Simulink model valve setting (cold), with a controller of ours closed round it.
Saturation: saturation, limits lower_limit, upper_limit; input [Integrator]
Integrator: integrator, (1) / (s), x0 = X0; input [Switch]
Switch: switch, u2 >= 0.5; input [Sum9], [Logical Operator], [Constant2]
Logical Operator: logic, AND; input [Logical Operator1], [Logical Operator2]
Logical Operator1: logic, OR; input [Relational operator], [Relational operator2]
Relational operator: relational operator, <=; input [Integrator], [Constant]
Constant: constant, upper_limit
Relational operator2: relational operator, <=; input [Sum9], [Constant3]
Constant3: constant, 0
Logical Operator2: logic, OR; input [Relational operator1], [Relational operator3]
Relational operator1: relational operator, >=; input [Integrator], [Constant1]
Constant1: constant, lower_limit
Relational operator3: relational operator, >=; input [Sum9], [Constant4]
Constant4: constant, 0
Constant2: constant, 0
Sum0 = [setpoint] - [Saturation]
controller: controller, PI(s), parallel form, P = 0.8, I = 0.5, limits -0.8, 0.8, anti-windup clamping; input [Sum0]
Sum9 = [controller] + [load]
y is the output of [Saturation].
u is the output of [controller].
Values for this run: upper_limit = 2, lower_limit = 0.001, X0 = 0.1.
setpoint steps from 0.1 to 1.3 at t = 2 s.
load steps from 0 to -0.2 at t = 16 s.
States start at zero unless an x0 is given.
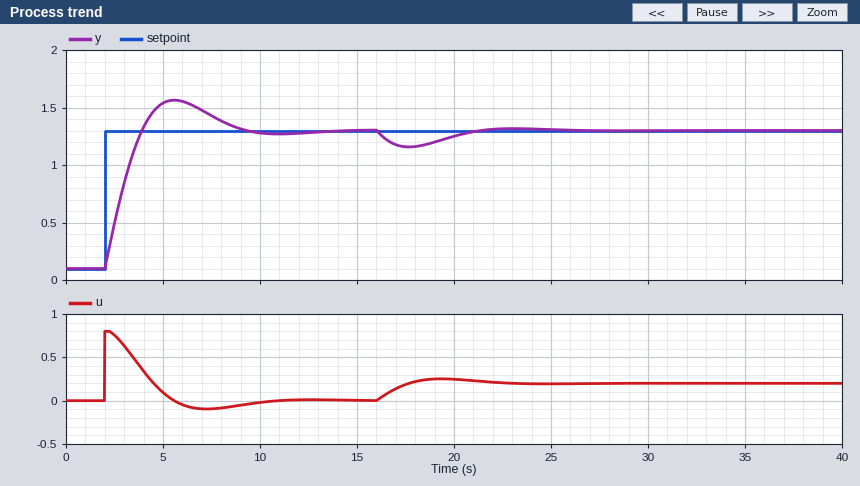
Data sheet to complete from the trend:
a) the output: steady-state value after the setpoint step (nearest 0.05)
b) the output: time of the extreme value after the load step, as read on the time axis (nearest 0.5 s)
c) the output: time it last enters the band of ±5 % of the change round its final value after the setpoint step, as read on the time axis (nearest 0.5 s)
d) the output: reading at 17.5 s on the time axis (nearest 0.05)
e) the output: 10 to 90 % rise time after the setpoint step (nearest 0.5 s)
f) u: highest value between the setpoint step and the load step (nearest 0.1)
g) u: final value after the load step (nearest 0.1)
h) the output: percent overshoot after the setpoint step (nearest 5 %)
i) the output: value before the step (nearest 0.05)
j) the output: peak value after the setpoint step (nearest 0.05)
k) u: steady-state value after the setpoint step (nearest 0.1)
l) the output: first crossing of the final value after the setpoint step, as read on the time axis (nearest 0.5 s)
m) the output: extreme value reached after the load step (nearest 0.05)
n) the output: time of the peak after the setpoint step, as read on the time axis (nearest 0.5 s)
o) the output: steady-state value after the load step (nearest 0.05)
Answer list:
1.30
17.5 s
8.5 s
1.15
1.5 s
0.8
0.2
20 %
0.10
1.55
0.0
4.0 s
1.15
5.5 s
1.30
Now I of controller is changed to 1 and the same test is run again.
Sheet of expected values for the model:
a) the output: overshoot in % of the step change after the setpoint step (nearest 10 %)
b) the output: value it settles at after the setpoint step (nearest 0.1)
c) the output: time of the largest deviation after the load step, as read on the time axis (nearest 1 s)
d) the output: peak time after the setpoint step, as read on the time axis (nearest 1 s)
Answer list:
30 %
1.3
17 s
5 s
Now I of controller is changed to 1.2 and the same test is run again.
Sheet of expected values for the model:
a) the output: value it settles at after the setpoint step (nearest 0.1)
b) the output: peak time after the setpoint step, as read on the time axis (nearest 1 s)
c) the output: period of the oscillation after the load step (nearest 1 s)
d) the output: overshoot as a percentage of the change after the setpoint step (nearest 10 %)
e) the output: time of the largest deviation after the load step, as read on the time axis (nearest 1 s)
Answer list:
1.3
5 s
6 s
30 %
17 s
